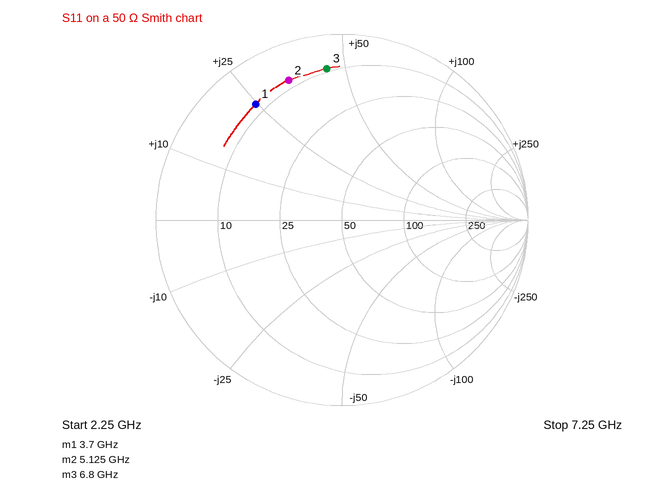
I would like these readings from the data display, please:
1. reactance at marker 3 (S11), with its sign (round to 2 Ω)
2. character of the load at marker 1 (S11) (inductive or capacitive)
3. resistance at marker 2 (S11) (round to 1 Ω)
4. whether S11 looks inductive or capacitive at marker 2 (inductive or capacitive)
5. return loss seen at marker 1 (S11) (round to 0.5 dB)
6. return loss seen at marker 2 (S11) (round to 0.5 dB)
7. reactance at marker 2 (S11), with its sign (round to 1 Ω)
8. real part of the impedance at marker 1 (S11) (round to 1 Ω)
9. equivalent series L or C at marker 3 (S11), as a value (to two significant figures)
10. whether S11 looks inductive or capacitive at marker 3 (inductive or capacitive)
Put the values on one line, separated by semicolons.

+44 Ω; inductive; 8 Ω; inductive; 2.0 dB; 2.0 dB; +34 Ω; 8 Ω; 1.0 nH; inductive
